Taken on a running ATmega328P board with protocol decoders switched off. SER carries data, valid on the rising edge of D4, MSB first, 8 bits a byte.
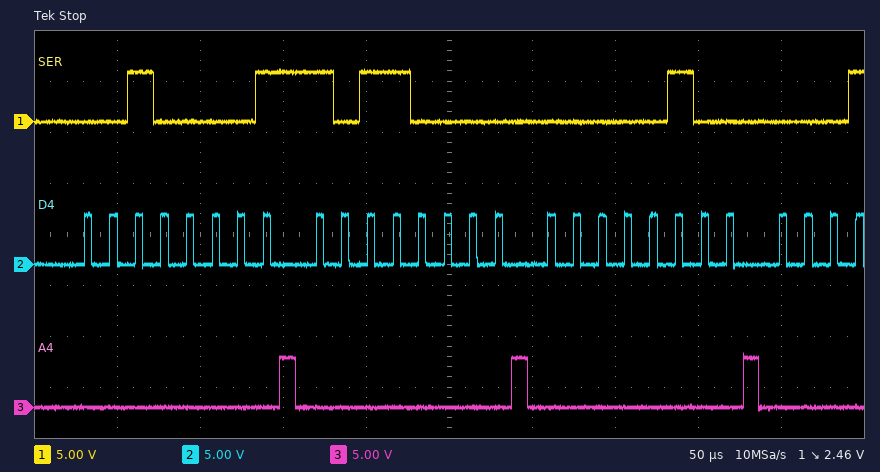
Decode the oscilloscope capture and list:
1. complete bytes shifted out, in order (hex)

21 B0 04
